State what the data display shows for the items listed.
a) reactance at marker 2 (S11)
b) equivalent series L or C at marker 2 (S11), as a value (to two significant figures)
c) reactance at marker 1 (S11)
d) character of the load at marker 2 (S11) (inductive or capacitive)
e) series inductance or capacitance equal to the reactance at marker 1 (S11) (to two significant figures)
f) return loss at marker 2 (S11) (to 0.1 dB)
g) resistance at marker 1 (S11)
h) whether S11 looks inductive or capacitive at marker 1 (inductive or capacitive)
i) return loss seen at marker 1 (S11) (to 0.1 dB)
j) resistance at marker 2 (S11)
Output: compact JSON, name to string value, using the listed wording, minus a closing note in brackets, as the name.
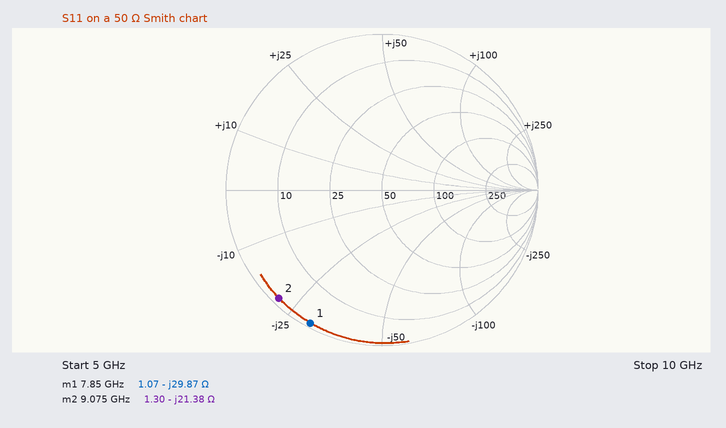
{"reactance at marker 2": "-21.38 Ω", "equivalent series L or C at marker 2 (S11), as a value": "820 fF", "reactance at marker 1": "-29.87 Ω", "character of the load at marker 2 (S11)": "capacitive", "series inductance or capacitance equal to the reactance at marker 1 (S11)": "680 fF", "return loss at marker 2 (S11)": "0.4 dB", "resistance at marker 1": "1.07 Ω", "whether S11 looks inductive or capacitive at marker 1": "capacitive", "return loss seen at marker 1 (S11)": "0.3 dB", "resistance at marker 2": "1.30 Ω"}
